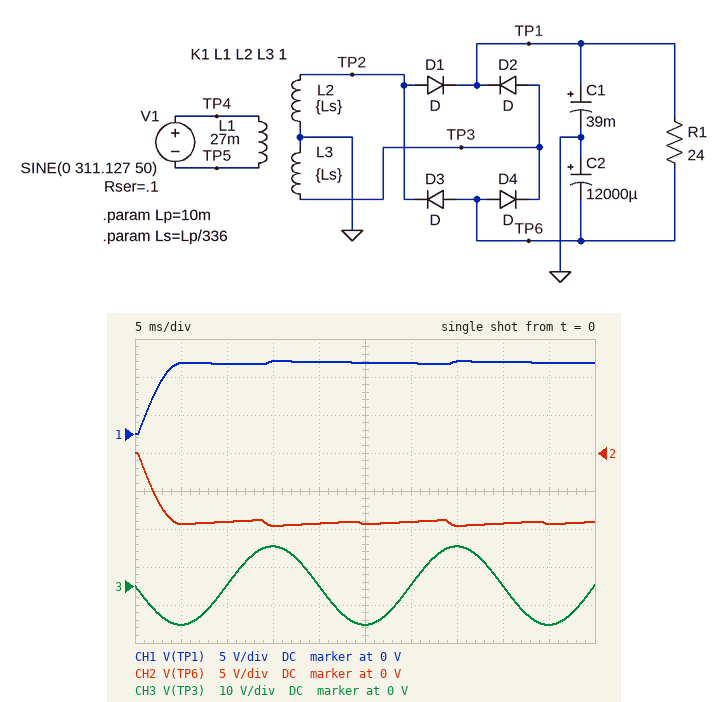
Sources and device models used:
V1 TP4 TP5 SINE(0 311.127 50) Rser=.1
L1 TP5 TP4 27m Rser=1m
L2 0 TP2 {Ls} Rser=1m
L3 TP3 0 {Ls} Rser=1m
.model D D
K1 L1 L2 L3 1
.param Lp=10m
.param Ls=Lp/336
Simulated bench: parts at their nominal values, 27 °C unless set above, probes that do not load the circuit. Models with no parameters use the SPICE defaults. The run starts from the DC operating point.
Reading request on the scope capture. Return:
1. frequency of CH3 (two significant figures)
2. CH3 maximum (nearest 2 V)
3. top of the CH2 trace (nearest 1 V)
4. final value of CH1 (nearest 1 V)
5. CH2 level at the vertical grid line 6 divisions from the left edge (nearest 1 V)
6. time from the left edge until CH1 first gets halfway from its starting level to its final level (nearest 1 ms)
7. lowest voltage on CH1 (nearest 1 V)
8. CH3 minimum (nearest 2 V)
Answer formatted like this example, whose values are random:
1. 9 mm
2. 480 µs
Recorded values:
1. 50 Hz
2. 10 V
3. 0 V
4. 9 V
5. -9 V
6. 2 ms
7. 0 V
8. -10 V
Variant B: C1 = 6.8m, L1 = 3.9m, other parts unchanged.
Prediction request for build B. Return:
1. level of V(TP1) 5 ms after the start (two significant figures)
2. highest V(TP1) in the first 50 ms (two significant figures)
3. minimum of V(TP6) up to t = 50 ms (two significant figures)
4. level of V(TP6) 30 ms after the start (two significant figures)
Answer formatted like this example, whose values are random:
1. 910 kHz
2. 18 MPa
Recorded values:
1. 24 V
2. 28 V
3. -28 V
4. -25 V
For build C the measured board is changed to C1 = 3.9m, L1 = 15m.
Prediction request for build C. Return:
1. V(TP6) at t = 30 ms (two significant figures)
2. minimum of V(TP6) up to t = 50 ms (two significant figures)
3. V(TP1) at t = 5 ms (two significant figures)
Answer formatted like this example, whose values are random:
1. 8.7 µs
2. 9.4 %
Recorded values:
1. -12 V
2. -13 V
3. 13 V
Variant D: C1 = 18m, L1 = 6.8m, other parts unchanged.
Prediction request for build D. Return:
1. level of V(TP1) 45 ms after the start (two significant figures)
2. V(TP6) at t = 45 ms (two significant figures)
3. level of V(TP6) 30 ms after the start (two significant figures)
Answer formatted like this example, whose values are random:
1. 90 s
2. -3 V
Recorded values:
1. 19 V
2. -19 V
3. -18 V
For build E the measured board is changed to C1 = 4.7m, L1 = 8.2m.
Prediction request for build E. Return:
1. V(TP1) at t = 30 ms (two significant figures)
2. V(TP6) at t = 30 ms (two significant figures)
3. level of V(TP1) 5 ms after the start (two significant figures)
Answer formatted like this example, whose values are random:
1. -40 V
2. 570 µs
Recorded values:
1. 16 V
2. -17 V
3. 17 V
